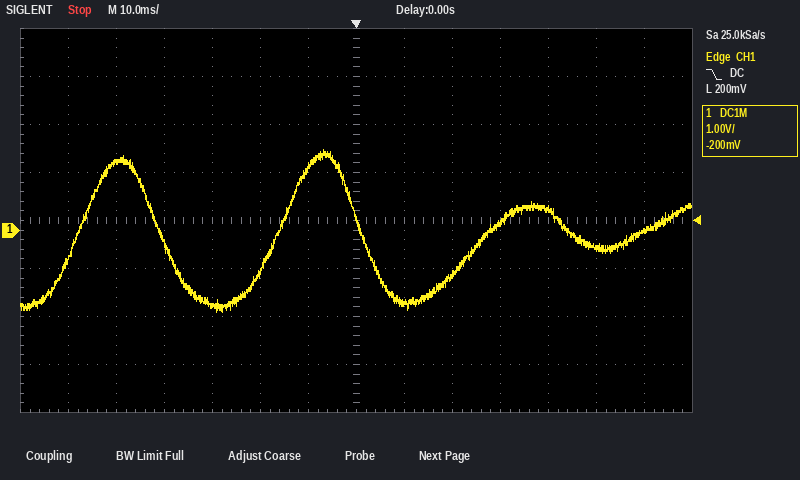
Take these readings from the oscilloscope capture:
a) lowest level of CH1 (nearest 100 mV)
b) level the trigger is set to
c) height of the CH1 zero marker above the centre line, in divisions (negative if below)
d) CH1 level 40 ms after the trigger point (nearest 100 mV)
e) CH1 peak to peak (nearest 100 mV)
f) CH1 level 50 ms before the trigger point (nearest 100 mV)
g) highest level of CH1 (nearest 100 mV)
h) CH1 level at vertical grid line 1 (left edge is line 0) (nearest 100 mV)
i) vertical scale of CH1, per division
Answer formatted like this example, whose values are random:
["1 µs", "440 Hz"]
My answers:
["-1.7 V", "200 mV", "-0.2 div", "400 mV", "3.4 V", "1.4 V", "1.7 V", "-600 mV", "1 V"]
